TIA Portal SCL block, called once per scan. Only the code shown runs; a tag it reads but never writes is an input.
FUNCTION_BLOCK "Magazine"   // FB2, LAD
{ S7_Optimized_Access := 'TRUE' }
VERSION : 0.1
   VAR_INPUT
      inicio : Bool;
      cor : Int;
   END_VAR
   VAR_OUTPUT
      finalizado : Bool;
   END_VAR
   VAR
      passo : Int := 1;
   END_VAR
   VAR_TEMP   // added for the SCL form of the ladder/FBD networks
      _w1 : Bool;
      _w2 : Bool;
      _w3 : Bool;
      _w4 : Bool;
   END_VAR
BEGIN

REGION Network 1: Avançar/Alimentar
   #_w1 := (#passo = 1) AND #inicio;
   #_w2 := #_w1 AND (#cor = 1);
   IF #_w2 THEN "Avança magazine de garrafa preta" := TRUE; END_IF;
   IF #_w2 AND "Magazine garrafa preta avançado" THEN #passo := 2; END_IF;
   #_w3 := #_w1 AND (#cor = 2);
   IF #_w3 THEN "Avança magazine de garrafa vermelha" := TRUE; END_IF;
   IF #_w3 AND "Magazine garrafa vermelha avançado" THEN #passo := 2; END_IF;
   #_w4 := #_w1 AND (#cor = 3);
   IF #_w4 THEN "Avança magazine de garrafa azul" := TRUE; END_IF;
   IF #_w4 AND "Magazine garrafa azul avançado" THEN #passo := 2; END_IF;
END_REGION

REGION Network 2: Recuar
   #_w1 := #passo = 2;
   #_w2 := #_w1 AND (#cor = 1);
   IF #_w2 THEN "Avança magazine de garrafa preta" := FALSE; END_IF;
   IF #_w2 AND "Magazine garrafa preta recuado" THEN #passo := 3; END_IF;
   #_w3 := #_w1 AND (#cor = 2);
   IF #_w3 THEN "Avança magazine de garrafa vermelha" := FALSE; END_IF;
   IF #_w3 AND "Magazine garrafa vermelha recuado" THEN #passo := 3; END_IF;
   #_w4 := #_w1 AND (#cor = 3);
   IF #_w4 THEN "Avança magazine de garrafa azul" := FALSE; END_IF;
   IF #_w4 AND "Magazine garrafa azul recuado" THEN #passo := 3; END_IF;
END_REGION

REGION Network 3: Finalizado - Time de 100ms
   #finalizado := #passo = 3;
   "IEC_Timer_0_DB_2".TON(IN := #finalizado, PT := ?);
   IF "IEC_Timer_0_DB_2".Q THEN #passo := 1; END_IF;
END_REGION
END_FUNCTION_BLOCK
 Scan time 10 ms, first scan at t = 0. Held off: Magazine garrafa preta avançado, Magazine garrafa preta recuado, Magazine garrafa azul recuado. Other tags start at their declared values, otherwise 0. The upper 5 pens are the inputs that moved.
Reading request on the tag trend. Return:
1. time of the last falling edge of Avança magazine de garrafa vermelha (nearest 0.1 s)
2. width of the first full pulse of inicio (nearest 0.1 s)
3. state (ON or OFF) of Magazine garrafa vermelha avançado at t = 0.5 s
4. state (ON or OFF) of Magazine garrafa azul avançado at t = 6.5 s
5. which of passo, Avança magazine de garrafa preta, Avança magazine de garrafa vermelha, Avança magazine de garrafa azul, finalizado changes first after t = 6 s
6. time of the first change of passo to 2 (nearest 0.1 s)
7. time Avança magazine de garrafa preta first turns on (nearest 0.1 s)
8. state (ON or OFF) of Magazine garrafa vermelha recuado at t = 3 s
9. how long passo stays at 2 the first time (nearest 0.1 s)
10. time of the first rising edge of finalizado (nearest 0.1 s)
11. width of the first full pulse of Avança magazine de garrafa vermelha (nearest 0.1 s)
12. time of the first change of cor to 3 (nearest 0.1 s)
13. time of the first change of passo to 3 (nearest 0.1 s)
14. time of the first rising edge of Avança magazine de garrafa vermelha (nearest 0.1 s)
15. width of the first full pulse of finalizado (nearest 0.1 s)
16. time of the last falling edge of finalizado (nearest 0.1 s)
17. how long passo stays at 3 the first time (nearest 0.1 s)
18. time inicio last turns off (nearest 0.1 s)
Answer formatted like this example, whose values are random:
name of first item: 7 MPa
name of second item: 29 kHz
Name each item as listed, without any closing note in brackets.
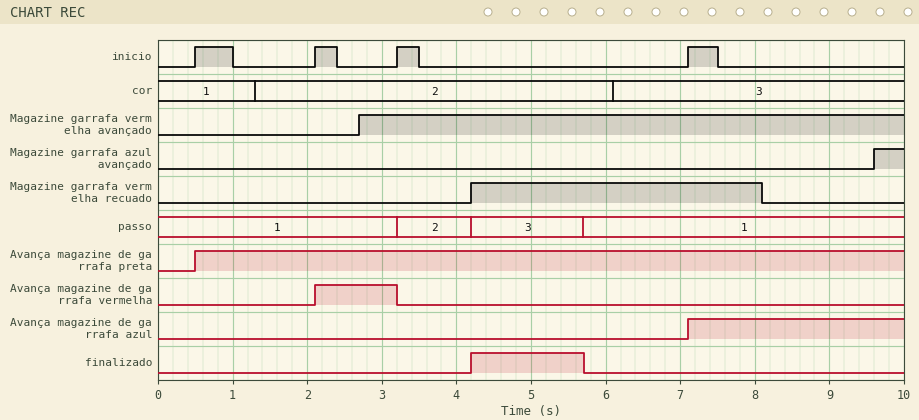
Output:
time of the last falling edge of Avança magazine de garrafa vermelha: 3.2 s
width of the first full pulse of inicio: 0.5 s
state (ON or OFF) of Magazine garrafa vermelha avançado at t = 0.5 s: OFF
state (ON or OFF) of Magazine garrafa azul avançado at t = 6.5 s: OFF
which of passo, Avança magazine de garrafa preta, Avança magazine de garrafa vermelha, Avança magazine de garrafa azul, finalizado changes first after t = 6 s: Avança magazine de garrafa azul
time of the first change of passo to 2: 3.2 s
time Avança magazine de garrafa preta first turns on: 0.5 s
state (ON or OFF) of Magazine garrafa vermelha recuado at t = 3 s: OFF
how long passo stays at 2 the first time: 1.0 s
time of the first rising edge of finalizado: 4.2 s
width of the first full pulse of Avança magazine de garrafa vermelha: 1.1 s
time of the first change of cor to 3: 6.1 s
time of the first change of passo to 3: 4.2 s
time of the first rising edge of Avança magazine de garrafa vermelha: 2.1 s
width of the first full pulse of finalizado: 1.5 s
time of the last falling edge of finalizado: 5.7 s
how long passo stays at 3 the first time: 1.5 s
time inicio last turns off: 7.5 s
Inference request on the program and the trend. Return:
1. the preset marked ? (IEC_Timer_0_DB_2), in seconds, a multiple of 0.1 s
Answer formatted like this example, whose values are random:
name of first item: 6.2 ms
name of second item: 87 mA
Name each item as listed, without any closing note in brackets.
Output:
the preset marked ? (IEC_Timer_0_DB_2), in seconds, a multiple of 0.1 s: 1.5 s
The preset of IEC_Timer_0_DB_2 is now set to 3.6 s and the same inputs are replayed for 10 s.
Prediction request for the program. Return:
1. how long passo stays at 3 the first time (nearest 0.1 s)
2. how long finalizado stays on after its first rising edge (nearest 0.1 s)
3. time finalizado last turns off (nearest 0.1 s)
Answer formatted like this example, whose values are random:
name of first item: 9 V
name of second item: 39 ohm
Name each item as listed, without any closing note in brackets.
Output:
how long passo stays at 3 the first time: 3.6 s
how long finalizado stays on after its first rising edge: 3.6 s
time finalizado last turns off: 7.8 s
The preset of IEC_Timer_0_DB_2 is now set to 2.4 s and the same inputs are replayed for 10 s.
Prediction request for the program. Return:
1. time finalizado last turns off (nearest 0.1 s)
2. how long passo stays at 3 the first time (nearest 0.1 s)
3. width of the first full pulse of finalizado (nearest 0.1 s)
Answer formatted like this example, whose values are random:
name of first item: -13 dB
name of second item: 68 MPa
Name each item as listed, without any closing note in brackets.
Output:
time finalizado last turns off: 6.6 s
how long passo stays at 3 the first time: 2.4 s
width of the first full pulse of finalizado: 2.4 s
